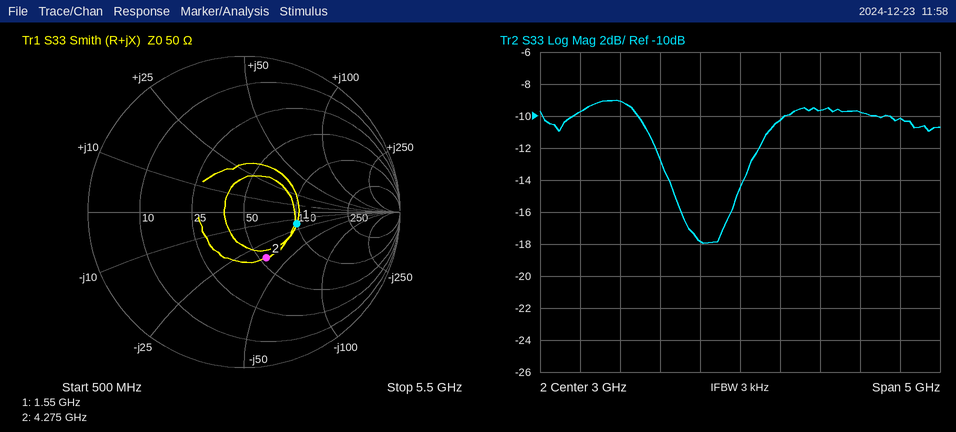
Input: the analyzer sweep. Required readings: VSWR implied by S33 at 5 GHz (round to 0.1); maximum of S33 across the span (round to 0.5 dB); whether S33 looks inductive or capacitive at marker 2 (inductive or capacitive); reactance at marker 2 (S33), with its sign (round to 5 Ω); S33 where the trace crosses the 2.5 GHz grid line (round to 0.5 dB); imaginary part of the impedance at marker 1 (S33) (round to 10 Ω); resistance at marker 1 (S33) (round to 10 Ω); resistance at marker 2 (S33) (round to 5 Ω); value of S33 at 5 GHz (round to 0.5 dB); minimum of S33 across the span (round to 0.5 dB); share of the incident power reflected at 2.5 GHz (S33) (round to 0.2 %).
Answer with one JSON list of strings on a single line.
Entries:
["1.9", "-9.0 dB", "capacitive", "-35 Ω", "-18.0 dB", "-20 Ω", "100 Ω", "55 Ω", "-10.0 dB", "-18.0 dB", "1.6 %"]
